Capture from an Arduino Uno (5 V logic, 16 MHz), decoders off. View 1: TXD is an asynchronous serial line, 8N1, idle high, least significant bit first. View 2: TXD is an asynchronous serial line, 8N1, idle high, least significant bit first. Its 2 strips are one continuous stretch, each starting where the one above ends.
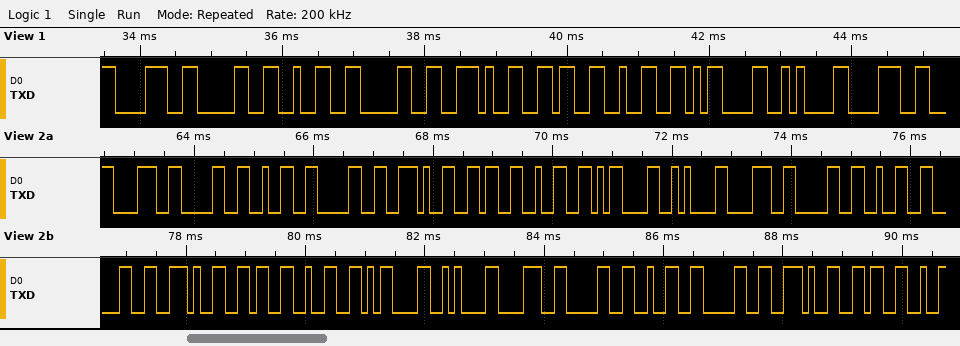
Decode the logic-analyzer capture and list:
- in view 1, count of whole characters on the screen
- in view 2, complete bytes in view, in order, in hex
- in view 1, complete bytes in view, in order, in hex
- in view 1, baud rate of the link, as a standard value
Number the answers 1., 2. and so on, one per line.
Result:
1. 10
2. 0x38 0x30 0x32 0x30 0x2E 0x36 0x32 0x0D 0x0A 0x38 0x30 0x32 0x30 0x2E 0x36 0x32 0x0D 0x0A 0x38 0x30 0x32 0x30 0x2E 0x36
3. 38 30 32 30 2E 36 32 0D 0A 38
4. 9600 baud
